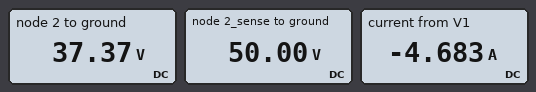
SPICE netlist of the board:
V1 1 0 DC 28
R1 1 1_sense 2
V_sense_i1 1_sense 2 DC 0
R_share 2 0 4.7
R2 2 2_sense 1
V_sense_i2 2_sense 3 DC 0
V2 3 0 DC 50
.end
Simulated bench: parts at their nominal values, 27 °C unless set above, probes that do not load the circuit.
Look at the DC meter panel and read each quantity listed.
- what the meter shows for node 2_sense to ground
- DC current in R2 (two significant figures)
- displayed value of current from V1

50.00 V
13 A
-4.683 A
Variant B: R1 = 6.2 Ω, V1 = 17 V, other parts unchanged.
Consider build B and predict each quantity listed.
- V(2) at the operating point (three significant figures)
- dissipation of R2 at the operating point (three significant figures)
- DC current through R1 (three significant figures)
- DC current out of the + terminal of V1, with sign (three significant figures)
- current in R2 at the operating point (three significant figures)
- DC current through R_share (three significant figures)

38.4 V
135 W
3.45 A
-3.45 A
11.6 A
8.17 A
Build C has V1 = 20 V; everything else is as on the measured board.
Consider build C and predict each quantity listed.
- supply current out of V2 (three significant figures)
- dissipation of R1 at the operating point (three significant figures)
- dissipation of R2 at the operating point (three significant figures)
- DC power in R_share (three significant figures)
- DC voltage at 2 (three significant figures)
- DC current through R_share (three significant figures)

15.0 A
113 W
224 W
261 W
35.0 V
7.45 A
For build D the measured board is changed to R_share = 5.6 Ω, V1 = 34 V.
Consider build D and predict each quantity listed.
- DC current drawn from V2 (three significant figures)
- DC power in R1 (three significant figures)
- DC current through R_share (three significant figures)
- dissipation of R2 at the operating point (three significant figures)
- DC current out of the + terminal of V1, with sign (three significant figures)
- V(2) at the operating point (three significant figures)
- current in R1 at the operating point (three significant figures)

10.1 A
17.5 W
7.13 A
102 W
-2.96 A
39.9 V
2.96 A
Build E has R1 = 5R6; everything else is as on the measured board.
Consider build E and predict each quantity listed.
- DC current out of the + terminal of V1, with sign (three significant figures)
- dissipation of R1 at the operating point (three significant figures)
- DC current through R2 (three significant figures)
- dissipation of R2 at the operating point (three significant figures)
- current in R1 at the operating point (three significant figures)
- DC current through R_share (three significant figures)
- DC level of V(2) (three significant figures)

-2.06 A
23.7 W
10.5 A
110 W
2.06 A
8.41 A
39.5 V
